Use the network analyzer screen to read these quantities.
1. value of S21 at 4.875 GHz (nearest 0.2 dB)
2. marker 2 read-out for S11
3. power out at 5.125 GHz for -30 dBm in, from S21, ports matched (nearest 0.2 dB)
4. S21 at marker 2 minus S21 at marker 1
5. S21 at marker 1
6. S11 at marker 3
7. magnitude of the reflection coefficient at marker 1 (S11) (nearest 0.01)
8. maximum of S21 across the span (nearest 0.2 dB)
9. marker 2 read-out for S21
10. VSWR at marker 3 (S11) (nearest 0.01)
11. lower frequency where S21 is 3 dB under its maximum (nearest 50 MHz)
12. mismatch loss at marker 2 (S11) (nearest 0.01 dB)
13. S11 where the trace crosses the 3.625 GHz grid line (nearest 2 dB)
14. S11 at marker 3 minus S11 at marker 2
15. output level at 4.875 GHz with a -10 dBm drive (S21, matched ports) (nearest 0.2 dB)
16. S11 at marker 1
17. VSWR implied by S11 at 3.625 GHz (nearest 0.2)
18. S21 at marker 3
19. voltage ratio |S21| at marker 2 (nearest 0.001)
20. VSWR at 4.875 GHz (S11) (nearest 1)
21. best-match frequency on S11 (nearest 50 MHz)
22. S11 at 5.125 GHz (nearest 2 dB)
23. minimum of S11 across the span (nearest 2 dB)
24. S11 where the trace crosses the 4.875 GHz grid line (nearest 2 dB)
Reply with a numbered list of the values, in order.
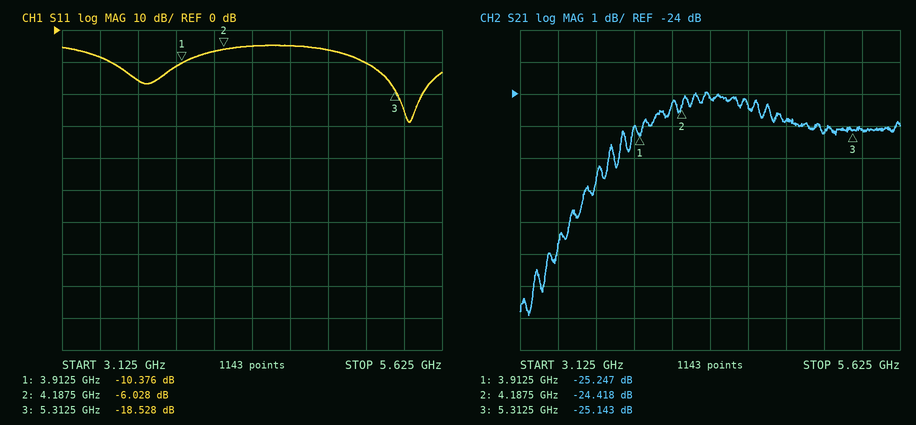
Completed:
1. -24.8 dB
2. -6.028 dB
3. -55.2 dBm
4. 0.829 dB
5. -25.247 dB
6. -18.528 dB
7. 0.30
8. -24.0 dB
9. -24.418 dB
10. 1.27
11. 3.60 GHz
12. 1.25 dB
13. -16 dB
14. -12.500 dB
15. -34.8 dBm
16. -10.376 dB
17. 1.4
18. -25.143 dB
19. 0.060
20. 3
21. 5.40 GHz
22. -10 dB
23. -28 dB
24. -6 dB
